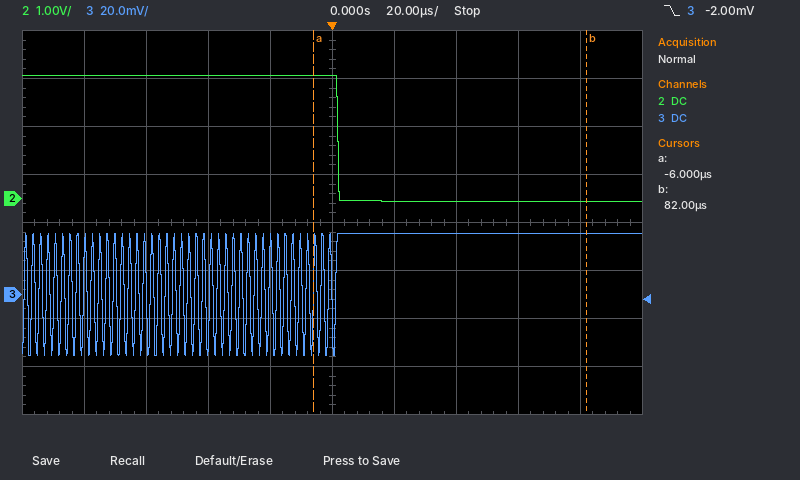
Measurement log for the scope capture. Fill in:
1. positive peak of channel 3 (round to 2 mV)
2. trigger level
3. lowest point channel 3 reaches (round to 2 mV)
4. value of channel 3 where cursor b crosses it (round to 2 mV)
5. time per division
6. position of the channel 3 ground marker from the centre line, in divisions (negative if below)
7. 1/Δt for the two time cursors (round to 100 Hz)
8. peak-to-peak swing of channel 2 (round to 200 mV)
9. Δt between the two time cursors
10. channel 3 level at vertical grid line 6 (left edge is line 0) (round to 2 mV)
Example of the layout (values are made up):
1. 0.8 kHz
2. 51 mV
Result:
1. 26 mV
2. -2.00 mV
3. -26 mV
4. 26 mV
5. 20 µs
6. -1.5 div
7. 11.4 kHz
8. 2.6 V
9. 88 µs
10. 26 mV
